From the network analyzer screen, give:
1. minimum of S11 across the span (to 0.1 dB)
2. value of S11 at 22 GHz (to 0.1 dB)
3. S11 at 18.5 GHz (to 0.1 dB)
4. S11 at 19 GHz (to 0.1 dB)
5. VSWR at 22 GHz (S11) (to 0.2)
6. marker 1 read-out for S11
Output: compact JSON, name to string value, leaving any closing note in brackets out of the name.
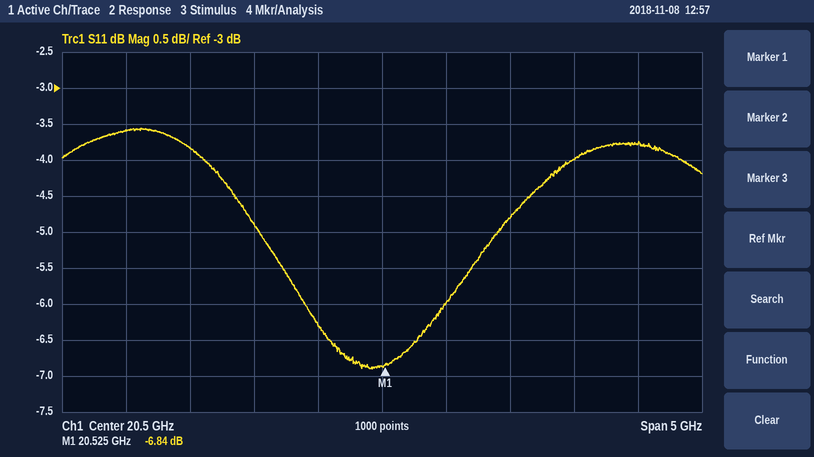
{"minimum of S11 across the span": "-6.9 dB", "value of S11 at 22 GHz": "-4.0 dB", "S11 at 18.5 GHz": "-3.6 dB", "S11 at 19 GHz": "-3.8 dB", "VSWR at 22 GHz (S11)": "4.4", "marker 1 read-out for S11": "-6.84 dB"}
